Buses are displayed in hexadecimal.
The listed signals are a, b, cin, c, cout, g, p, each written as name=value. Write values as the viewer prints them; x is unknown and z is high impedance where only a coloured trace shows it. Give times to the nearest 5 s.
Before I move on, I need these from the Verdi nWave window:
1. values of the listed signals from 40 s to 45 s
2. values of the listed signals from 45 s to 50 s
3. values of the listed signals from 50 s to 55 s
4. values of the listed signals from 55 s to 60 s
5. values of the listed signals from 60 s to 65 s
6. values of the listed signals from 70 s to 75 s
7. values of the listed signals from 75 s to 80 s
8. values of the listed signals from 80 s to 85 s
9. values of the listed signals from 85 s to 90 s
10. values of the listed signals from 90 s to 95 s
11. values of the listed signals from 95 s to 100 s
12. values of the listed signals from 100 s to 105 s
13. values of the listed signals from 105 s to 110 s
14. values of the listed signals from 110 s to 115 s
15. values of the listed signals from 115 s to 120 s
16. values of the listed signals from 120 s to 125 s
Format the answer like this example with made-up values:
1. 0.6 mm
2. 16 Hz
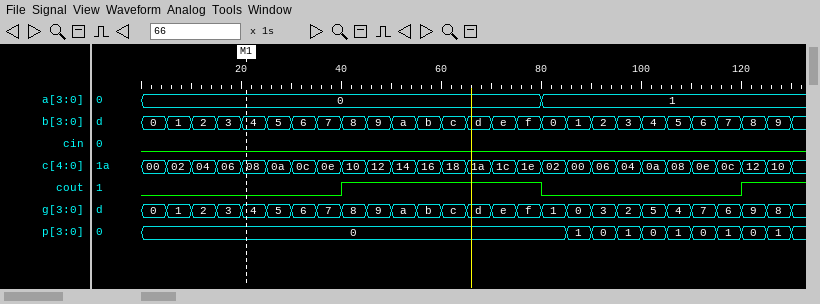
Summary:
1. a=0, b=8, cin=0, c=10, cout=1, g=8, p=0
2. a=0, b=9, cin=0, c=12, cout=1, g=9, p=0
3. a=0, b=a, cin=0, c=14, cout=1, g=a, p=0
4. a=0, b=b, cin=0, c=16, cout=1, g=b, p=0
5. a=0, b=c, cin=0, c=18, cout=1, g=c, p=0
6. a=0, b=e, cin=0, c=1c, cout=1, g=e, p=0
7. a=0, b=f, cin=0, c=1e, cout=1, g=f, p=0
8. a=1, b=0, cin=0, c=02, cout=0, g=1, p=0
9. a=1, b=1, cin=0, c=00, cout=0, g=0, p=1
10. a=1, b=2, cin=0, c=06, cout=0, g=3, p=0
11. a=1, b=3, cin=0, c=04, cout=0, g=2, p=1
12. a=1, b=4, cin=0, c=0a, cout=0, g=5, p=0
13. a=1, b=5, cin=0, c=08, cout=0, g=4, p=1
14. a=1, b=6, cin=0, c=0e, cout=0, g=7, p=0
15. a=1, b=7, cin=0, c=0c, cout=0, g=6, p=1
16. a=1, b=8, cin=0, c=12, cout=1, g=9, p=0
